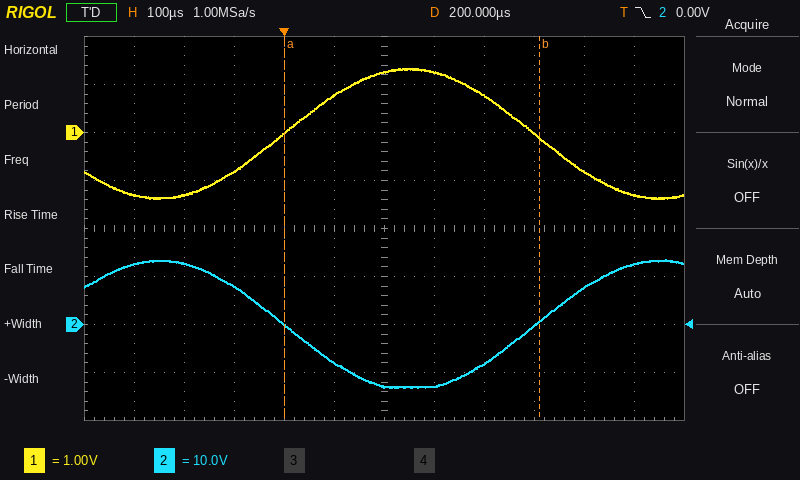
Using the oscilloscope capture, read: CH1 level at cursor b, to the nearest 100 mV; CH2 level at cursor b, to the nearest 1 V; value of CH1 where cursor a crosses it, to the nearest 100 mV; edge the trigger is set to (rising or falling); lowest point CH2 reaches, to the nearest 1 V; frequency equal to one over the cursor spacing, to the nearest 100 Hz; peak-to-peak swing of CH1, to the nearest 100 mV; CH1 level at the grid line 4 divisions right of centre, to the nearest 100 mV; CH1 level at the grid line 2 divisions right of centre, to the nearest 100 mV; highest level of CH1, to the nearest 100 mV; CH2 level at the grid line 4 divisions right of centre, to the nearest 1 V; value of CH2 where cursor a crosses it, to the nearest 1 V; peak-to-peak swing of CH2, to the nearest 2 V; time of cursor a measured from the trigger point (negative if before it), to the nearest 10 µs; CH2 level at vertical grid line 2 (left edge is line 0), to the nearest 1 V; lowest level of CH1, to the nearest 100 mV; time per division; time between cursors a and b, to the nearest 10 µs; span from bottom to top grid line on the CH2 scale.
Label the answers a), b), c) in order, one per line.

a) -100 mV
b) 1 V
c) 0.0 V
d) falling
e) -13 V
f) 2.0 kHz
g) 2.7 V
h) -800 mV
i) 800 mV
j) 1.3 V
k) 8 V
l) 0 V
m) 26 V
n) 0 µs
o) 13 V
p) -1.4 V
q) 100 µs
r) 510 µs
s) 80 V
